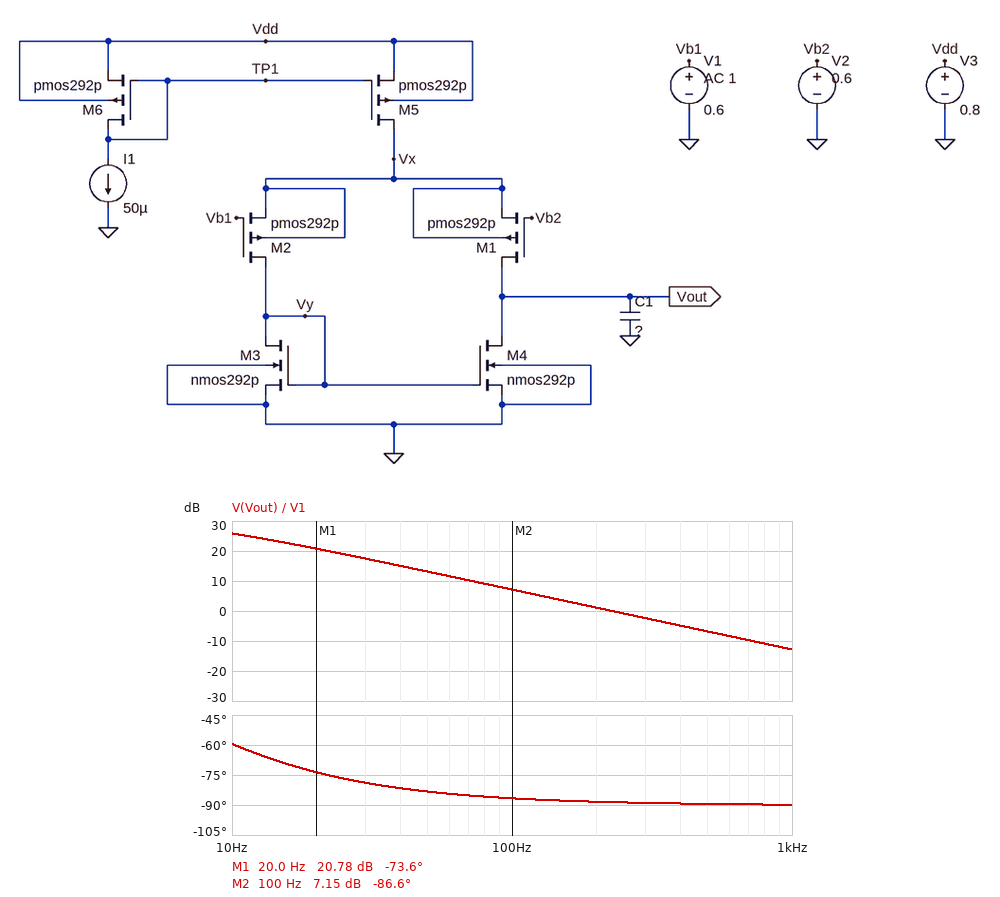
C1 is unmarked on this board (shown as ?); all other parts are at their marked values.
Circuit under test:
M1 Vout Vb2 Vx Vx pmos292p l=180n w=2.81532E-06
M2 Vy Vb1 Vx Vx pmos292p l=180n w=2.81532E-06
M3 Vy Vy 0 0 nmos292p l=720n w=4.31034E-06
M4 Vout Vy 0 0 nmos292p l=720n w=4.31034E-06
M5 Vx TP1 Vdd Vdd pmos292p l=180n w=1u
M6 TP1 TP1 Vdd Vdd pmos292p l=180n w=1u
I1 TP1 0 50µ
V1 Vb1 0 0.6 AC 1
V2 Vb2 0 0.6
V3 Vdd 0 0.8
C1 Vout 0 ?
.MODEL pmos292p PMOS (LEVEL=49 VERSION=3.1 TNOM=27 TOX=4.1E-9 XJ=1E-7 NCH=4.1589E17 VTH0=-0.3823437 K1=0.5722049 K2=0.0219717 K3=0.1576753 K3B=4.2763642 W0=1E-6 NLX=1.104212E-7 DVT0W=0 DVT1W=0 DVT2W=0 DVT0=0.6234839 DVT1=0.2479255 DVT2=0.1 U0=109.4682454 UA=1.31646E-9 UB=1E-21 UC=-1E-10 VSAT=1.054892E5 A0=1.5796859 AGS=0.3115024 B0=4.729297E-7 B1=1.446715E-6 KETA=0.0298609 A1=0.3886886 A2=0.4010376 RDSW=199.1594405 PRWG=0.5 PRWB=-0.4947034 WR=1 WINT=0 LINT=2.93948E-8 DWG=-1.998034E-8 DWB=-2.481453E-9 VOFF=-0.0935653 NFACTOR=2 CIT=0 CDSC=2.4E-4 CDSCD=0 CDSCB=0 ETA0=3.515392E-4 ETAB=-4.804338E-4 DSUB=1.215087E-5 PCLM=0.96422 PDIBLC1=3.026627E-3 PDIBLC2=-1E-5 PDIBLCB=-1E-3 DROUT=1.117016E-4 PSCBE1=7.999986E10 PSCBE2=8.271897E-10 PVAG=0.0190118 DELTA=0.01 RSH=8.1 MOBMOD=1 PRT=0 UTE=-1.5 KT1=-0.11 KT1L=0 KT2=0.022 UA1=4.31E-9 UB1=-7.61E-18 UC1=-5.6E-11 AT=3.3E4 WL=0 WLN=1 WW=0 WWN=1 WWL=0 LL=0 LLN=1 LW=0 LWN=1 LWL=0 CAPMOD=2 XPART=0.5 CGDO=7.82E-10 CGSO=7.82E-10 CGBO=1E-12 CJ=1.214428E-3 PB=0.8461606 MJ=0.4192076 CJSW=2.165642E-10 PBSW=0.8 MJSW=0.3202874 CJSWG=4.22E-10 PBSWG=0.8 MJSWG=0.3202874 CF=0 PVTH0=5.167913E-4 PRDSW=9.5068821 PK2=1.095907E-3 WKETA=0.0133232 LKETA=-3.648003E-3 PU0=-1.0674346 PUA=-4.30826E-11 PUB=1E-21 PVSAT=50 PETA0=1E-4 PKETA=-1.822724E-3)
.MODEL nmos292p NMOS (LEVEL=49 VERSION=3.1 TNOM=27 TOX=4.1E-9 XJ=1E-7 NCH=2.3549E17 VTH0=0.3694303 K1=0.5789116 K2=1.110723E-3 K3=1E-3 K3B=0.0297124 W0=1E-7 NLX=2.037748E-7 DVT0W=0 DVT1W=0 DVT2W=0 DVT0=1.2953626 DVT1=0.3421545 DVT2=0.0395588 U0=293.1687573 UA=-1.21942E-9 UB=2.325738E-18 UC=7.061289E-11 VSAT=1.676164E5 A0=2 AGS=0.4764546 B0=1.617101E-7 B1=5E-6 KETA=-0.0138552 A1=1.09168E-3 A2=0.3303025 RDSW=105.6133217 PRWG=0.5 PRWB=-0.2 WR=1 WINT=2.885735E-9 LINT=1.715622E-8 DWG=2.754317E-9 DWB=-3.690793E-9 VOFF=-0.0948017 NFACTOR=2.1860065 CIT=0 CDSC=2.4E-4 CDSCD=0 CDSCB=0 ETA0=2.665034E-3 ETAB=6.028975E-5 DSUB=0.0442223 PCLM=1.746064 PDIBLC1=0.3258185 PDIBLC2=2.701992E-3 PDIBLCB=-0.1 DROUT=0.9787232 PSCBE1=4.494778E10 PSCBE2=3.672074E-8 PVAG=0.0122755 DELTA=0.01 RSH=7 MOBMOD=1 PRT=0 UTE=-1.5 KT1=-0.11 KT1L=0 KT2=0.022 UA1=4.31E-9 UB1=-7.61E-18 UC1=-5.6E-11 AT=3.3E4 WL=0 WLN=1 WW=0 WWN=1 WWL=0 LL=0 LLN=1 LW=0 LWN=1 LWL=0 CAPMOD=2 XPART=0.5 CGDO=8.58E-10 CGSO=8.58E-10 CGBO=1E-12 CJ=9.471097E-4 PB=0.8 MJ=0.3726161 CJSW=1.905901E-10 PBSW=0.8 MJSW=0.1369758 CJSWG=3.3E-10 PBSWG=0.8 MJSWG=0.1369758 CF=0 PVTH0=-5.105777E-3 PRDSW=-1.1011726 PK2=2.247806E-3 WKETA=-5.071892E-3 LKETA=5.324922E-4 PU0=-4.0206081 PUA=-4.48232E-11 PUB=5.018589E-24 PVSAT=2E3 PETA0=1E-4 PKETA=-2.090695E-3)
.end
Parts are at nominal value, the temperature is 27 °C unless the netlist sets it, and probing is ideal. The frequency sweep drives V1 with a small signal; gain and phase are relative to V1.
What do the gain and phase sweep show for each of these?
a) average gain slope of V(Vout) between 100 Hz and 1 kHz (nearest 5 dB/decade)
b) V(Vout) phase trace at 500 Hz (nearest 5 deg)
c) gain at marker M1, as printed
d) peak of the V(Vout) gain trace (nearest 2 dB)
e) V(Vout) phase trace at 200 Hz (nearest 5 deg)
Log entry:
-20 dB/decade
-90 deg
20.78 dB
26 dB
-90 deg
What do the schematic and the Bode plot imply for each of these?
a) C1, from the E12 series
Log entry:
33 pF
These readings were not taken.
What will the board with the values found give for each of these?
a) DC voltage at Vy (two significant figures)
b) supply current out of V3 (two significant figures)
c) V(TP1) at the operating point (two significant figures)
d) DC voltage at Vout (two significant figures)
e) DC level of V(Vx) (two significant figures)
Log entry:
190 mV
50 µA
-150 mV
190 mV
800 mV
